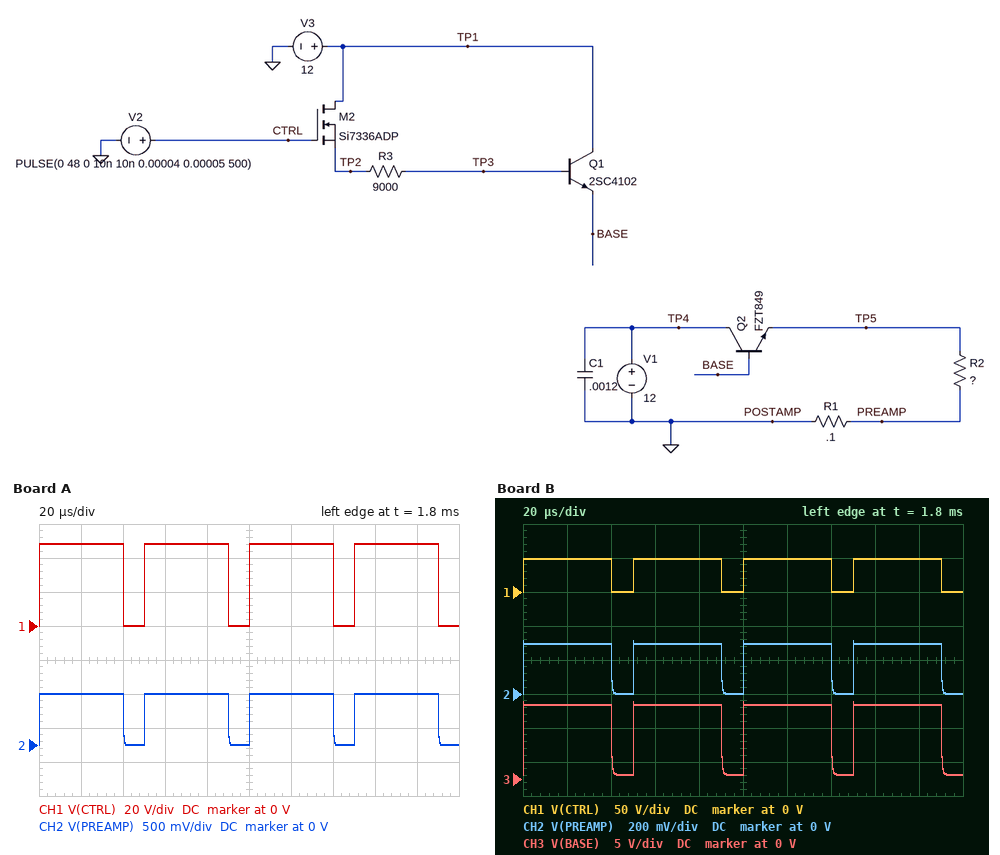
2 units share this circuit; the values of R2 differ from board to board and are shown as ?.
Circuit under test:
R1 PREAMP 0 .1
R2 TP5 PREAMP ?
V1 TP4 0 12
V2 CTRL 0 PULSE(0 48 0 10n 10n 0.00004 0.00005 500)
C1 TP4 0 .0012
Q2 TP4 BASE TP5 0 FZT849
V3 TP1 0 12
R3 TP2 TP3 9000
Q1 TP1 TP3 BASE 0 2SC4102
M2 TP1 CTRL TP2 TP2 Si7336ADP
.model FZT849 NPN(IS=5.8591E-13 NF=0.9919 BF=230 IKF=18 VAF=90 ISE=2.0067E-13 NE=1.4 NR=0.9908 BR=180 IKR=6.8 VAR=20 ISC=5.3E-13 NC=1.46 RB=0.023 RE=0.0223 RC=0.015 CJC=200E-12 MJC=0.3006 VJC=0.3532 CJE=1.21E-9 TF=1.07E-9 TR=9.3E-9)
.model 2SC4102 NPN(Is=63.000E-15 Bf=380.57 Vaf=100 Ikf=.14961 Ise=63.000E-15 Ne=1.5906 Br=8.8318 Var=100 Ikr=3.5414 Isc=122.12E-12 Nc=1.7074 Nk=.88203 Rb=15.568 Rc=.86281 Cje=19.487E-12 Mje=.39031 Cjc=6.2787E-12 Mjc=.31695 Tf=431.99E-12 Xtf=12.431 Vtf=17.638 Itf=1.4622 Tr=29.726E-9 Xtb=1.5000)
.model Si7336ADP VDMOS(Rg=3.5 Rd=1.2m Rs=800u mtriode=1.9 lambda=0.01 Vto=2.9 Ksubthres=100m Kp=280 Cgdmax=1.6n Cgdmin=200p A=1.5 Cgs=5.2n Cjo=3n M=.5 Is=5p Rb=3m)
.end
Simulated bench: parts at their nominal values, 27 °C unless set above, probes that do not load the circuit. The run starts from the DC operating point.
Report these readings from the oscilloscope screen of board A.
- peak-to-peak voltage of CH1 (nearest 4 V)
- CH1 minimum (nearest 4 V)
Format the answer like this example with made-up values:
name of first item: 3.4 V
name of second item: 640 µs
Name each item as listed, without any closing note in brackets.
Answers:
peak-to-peak voltage of CH1: 48 V
CH1 minimum: 0 V
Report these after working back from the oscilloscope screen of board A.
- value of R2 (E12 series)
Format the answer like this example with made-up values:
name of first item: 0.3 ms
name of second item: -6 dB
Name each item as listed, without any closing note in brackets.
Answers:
value of R2: 1 Ω
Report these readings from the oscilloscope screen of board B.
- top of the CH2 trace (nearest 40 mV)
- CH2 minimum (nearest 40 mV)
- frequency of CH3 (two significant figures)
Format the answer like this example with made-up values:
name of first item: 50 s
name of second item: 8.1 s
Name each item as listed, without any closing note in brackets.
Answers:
top of the CH2 trace: 320 mV
CH2 minimum: 0 V
frequency of CH3: 20 kHz
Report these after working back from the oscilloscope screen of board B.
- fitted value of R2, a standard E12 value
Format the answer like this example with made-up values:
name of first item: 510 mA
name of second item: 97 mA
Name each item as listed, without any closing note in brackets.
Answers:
fitted value of R2, a standard E12 value: 3.3 Ω
